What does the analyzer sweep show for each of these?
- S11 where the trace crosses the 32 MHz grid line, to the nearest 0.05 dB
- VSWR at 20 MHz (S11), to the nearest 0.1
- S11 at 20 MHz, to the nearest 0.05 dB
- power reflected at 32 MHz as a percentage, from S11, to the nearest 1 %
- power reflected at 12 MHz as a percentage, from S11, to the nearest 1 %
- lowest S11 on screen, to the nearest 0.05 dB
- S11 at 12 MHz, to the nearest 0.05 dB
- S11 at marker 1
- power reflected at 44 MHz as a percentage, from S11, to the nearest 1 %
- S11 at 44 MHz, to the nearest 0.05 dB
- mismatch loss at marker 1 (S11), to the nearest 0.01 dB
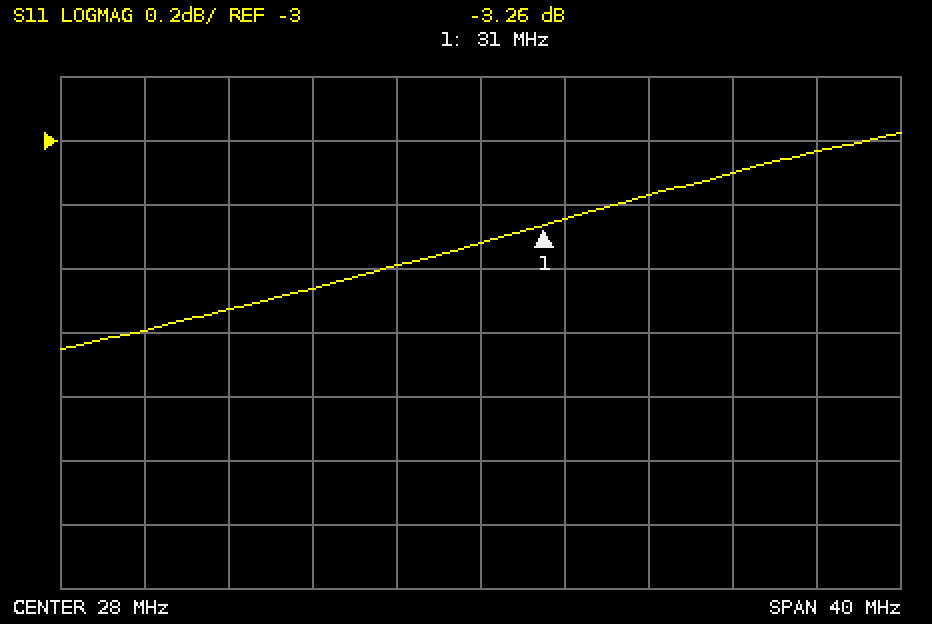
-3.25 dB
5.1
-3.45 dB
47 %
44 %
-3.65 dB
-3.60 dB
-3.26 dB
50 %
-3.05 dB
2.77 dB
